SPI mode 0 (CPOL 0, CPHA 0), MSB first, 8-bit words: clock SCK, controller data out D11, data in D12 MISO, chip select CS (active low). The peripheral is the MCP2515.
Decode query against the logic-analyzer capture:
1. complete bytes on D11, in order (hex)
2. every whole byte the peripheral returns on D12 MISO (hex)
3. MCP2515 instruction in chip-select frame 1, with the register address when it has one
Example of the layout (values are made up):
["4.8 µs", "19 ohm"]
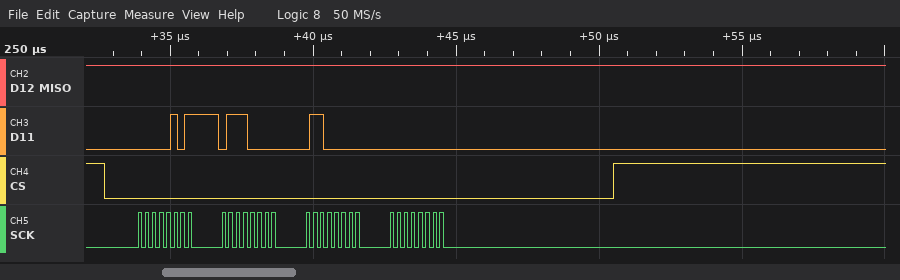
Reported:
["0x05 0x70 0x60 0x00", "0xFF 0xFF 0xFF 0xFF", "BIT MODIFY 0x70"]
